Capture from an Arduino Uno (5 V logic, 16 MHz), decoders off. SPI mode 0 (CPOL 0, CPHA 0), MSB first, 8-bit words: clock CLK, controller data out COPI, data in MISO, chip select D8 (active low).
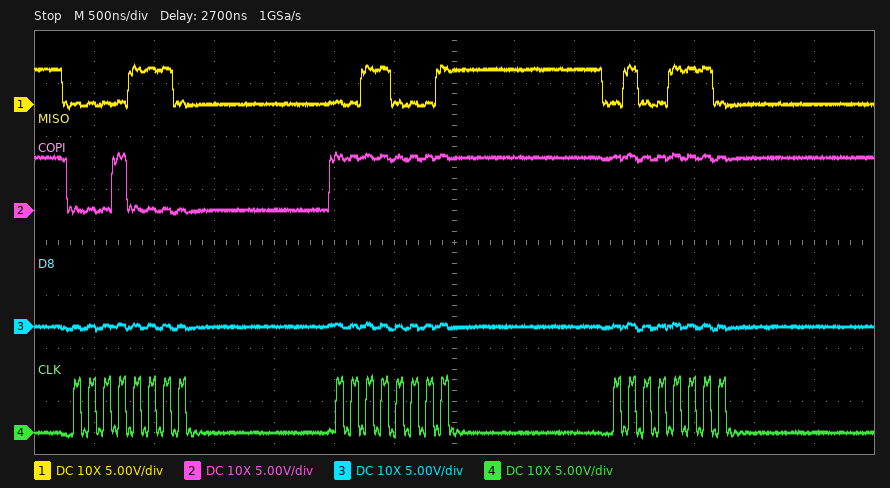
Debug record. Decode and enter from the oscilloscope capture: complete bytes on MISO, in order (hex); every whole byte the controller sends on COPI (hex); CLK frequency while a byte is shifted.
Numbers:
0E 31 4E
10 FF FF
8 MHz
